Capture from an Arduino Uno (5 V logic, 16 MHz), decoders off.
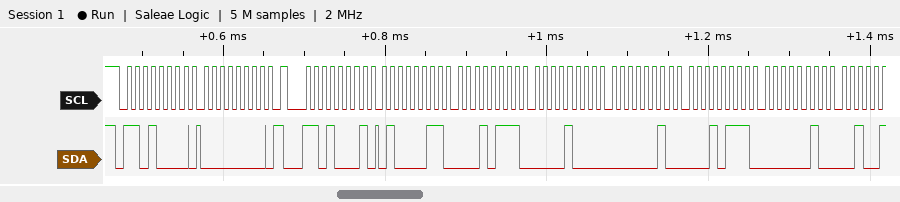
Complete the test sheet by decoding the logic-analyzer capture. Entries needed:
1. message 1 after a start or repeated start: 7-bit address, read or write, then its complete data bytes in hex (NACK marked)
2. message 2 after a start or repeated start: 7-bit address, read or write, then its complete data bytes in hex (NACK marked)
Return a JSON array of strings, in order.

["0x68 write: 00", "0x68 read: 43 17 08 02 17 02"]
